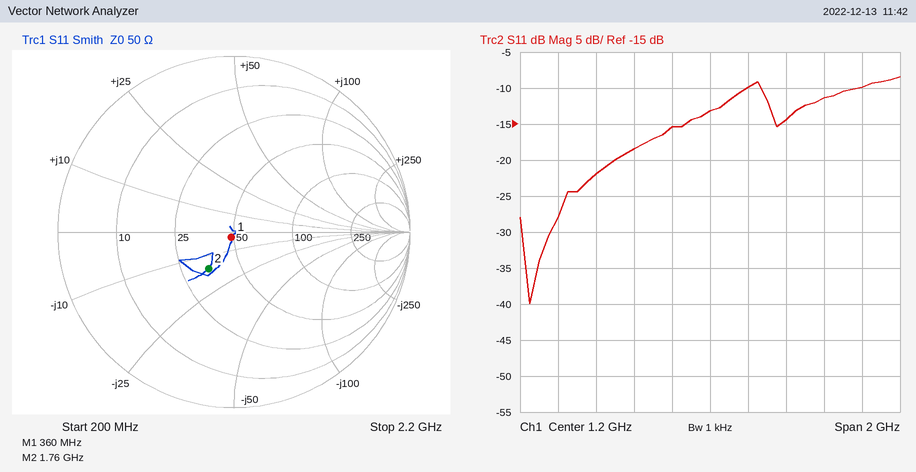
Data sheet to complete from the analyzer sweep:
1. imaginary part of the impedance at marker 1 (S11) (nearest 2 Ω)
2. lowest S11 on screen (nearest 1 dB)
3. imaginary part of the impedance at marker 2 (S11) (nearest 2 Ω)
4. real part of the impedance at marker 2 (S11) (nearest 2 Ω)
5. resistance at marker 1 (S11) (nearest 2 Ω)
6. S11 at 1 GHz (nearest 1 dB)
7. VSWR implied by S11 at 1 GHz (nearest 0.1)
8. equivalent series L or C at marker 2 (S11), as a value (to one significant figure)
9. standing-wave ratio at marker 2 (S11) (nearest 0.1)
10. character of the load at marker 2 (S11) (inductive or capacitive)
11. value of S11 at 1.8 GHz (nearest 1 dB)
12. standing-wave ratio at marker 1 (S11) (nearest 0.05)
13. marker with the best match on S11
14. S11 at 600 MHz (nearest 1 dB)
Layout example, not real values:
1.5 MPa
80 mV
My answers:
-2 Ω
-40 dB
-16 Ω
34 Ω
48 Ω
-15 dB
1.4
6 pF
1.7
capacitive
-11 dB
1.05
marker 1
-22 dB
